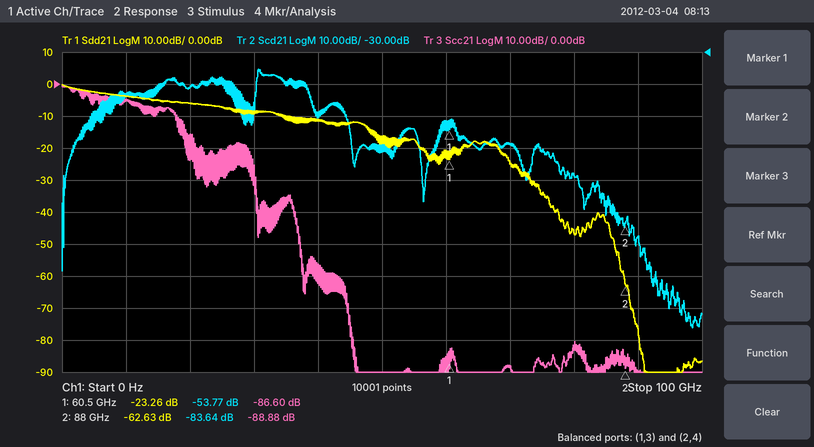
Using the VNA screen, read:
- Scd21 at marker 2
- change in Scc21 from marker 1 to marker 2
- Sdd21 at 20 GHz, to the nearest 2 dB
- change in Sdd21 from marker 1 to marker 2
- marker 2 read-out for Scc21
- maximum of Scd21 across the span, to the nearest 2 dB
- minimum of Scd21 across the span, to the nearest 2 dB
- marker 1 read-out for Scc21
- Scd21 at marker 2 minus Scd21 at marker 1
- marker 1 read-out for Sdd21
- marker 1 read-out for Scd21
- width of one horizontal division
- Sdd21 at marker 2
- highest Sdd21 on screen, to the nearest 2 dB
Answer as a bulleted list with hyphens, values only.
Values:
- -83.64 dB
- -2.28 dB
- -6 dB
- -39.37 dB
- -88.88 dB
- -36 dB
- -116 dB
- -86.60 dB
- -29.87 dB
- -23.26 dB
- -53.77 dB
- 10 GHz
- -62.63 dB
- 0 dB
